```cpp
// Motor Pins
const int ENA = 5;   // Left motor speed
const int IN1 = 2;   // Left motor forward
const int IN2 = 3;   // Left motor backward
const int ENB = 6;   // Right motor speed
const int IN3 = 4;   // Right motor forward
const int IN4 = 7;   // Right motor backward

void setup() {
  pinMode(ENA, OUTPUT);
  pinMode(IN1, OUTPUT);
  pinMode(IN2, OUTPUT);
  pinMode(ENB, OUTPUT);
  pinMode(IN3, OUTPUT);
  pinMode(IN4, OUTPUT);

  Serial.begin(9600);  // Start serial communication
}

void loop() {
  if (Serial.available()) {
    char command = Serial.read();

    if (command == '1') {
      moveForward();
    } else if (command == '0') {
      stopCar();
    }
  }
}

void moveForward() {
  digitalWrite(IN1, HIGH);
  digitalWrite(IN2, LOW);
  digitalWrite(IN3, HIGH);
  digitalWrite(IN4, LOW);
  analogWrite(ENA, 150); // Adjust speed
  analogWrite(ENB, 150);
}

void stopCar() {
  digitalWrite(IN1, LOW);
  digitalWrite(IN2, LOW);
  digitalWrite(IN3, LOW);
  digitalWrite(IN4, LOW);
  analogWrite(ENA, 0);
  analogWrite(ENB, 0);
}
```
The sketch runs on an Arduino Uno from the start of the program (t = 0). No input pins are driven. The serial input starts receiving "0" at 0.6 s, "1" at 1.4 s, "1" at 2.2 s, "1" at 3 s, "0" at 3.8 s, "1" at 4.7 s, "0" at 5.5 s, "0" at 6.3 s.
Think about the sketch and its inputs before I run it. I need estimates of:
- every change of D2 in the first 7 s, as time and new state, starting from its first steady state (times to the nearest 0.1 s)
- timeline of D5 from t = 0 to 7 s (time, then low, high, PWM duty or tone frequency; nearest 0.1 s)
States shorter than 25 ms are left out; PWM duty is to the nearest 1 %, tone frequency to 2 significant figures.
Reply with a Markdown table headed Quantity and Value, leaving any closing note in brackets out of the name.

| Quantity | Value |
|---|---|
| every change of D2 in the first 7 s, as time and new state, starting from its first steady state | 0 s low; 1.4 s high; 3.8 s low; 4.7 s high; 5.5 s low |
| timeline of D5 from t = 0 to 7 s | 0 s low; 1.4 s PWM 59 %; 3.8 s low; 4.7 s PWM 59 %; 5.5 s low |
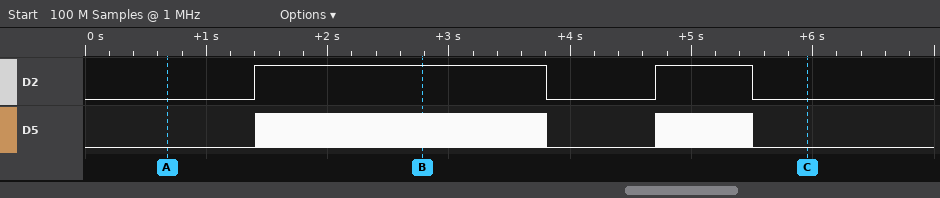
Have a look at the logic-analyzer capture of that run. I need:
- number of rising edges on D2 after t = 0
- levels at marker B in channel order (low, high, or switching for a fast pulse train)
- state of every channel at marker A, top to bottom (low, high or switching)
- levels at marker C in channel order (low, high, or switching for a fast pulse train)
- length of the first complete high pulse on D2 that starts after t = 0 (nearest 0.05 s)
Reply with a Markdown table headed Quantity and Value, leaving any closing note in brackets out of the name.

| Quantity | Value |
|---|---|
| number of rising edges on D2 after t = 0 | 2 |
| levels at marker B in channel order | D2 high, D5 switching |
| state of every channel at marker A, top to bottom | D2 low, D5 low |
| levels at marker C in channel order | D2 low, D5 low |
| length of the first complete high pulse on D2 that starts after t = 0 | 2.40 s |
